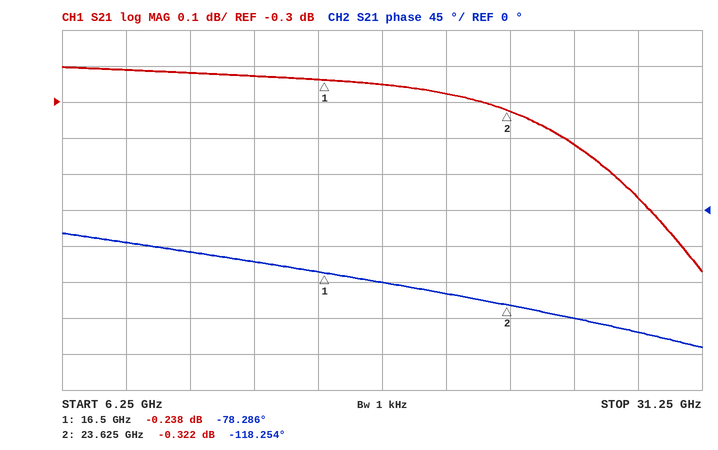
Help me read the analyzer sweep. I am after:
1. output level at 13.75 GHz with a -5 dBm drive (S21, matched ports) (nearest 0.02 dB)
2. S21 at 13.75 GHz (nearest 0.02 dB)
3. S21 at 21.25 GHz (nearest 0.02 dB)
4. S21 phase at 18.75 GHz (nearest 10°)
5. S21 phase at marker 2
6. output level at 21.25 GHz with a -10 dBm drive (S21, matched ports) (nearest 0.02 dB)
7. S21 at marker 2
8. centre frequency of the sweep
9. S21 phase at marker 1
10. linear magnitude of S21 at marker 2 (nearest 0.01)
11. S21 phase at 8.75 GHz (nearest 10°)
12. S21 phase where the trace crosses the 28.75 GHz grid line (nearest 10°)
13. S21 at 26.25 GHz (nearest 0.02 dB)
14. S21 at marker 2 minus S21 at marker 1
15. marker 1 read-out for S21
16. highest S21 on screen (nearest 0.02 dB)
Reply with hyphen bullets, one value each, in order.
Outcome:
- -5.22 dBm
- -0.22 dB
- -0.28 dB
- -90°
- -118.254°
- -10.28 dBm
- -0.322 dB
- 18.75 GHz
- -78.286°
- 0.96
- -40°
- -150°
- -0.42 dB
- -0.084 dB
- -0.238 dB
- -0.20 dB
